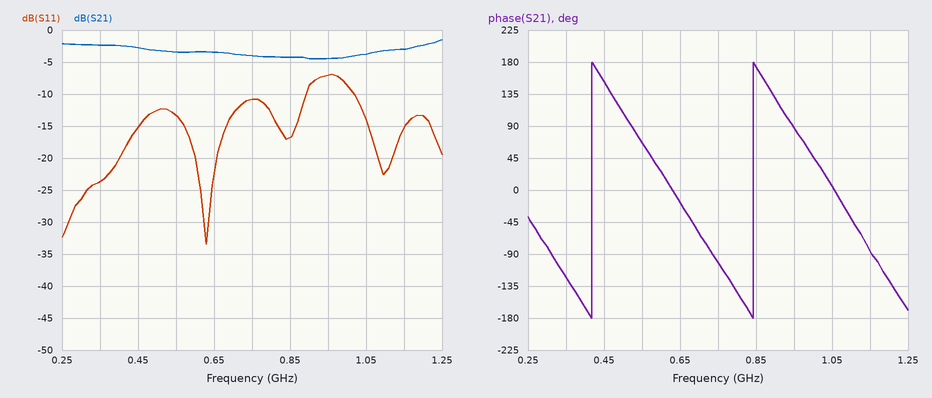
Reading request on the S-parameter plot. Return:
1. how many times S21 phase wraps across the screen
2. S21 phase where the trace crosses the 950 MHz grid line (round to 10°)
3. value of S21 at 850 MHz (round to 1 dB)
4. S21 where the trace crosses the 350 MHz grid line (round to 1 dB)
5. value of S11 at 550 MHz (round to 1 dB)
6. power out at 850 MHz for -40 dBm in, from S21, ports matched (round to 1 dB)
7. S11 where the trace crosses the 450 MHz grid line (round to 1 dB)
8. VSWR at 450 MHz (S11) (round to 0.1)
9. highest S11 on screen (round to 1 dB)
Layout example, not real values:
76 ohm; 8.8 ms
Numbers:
2; 90°; -4 dB; -2 dB; -13 dB; -44 dBm; -15 dB; 1.4; -7 dB
